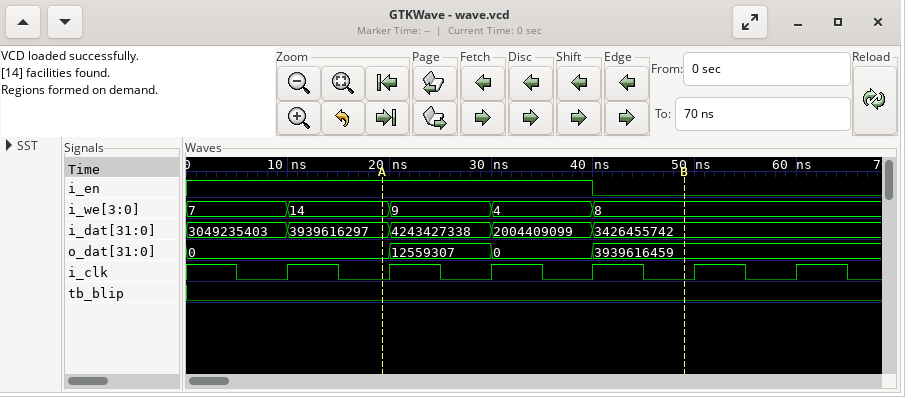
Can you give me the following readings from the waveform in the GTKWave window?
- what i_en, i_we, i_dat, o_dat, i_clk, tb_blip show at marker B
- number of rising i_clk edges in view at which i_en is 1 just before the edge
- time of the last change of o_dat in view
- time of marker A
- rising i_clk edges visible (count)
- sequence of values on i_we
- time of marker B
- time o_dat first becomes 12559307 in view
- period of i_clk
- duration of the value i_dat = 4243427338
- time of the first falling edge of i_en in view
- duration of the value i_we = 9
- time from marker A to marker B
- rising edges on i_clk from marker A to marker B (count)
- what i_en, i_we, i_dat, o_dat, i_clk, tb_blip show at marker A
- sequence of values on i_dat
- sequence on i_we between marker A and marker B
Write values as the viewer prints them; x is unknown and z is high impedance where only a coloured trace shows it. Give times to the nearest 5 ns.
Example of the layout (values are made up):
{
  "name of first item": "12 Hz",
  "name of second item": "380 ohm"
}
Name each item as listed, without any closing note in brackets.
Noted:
{
  "what i_en, i_we, i_dat, o_dat, i_clk, tb_blip show at marker B": "i_en=0, i_we=8, i_dat=3426455742, o_dat=3939616459, i_clk=0, tb_blip=0",
  "number of rising i_clk edges in view at which i_en is 1 just before the edge": "4",
  "time of the last change of o_dat in view": "40 ns",
  "time of marker A": "20 ns",
  "rising i_clk edges visible": "6",
  "sequence of values on i_we": "7, 14, 9, 4, 8",
  "time of marker B": "50 ns",
  "time o_dat first becomes 12559307 in view": "20 ns",
  "period of i_clk": "10 ns",
  "duration of the value i_dat = 4243427338": "10 ns",
  "time of the first falling edge of i_en in view": "40 ns",
  "duration of the value i_we = 9": "10 ns",
  "time from marker A to marker B": "30 ns",
  "rising edges on i_clk from marker A to marker B": "3",
  "what i_en, i_we, i_dat, o_dat, i_clk, tb_blip show at marker A": "i_en=1, i_we=14, i_dat=3939616297, o_dat=0, i_clk=0, tb_blip=0",
  "sequence of values on i_dat": "3049235403, 3939616297, 4243427338, 2004409099, 3426455742",
  "sequence on i_we between marker A and marker B": "14, 9, 4, 8"
}
